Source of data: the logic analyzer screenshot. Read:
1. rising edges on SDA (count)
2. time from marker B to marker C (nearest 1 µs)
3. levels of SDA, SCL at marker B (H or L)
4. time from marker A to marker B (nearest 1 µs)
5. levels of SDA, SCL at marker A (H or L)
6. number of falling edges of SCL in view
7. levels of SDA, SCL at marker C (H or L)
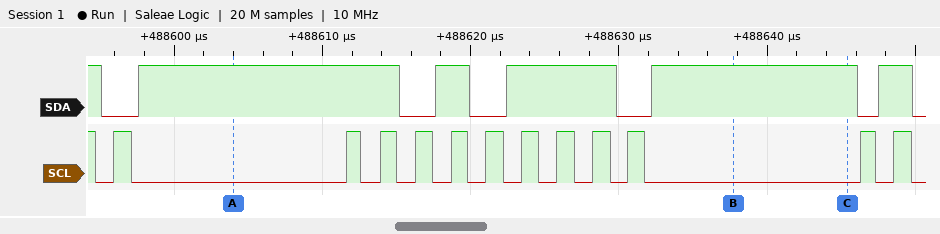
5
8 µs
SDA=H, SCL=L
34 µs
SDA=H, SCL=L
13
SDA=H, SCL=L
